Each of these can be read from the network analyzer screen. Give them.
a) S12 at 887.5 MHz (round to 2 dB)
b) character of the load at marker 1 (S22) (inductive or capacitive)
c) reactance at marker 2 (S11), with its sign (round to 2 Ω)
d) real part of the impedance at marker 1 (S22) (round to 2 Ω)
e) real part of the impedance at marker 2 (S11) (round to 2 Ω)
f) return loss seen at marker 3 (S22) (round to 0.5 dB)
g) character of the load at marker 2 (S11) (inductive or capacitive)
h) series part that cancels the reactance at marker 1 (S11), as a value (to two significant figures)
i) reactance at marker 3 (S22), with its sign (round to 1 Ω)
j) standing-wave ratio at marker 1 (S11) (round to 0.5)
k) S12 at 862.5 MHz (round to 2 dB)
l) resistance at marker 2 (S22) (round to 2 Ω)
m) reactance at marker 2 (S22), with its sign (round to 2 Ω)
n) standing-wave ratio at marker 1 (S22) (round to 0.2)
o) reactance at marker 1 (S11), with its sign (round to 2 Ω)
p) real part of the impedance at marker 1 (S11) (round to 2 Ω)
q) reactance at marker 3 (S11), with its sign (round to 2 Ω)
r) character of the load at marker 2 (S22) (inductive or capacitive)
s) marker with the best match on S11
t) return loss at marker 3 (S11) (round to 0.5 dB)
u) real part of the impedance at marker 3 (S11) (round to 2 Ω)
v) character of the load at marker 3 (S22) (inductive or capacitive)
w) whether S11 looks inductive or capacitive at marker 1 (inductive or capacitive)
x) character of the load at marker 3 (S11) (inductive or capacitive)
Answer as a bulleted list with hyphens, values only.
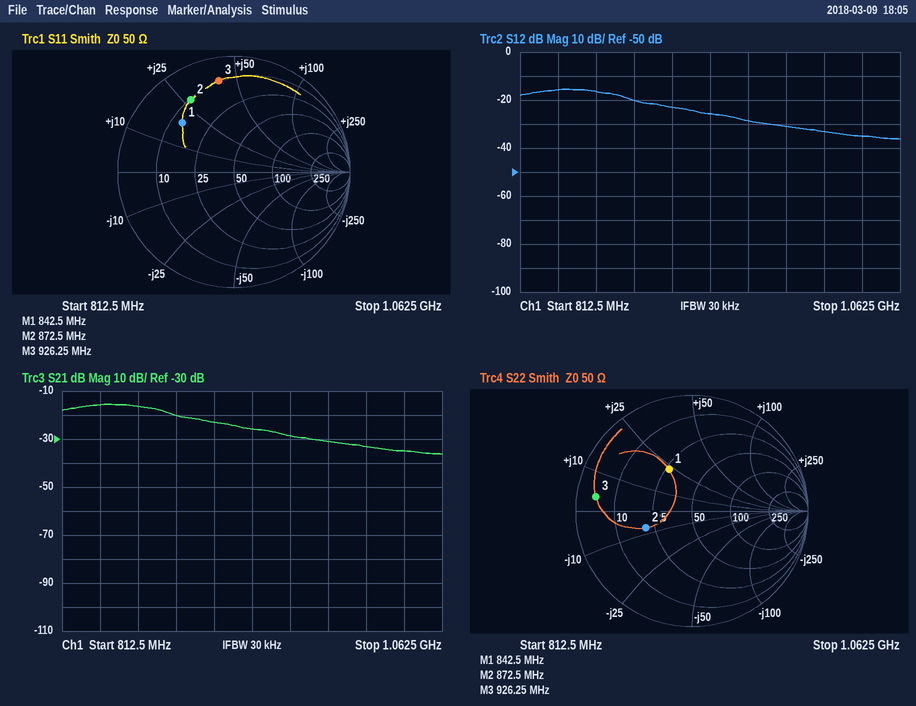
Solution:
- -20 dB
- inductive
- +28 Ω
- 26 Ω
- 10 Ω
- 1.5 dB
- inductive
- 10 pF
- +4 Ω
- 4.0
- -16 dB
- 20 Ω
- -8 Ω
- 2.4
- +18 Ω
- 14 Ω
- +42 Ω
- capacitive
- marker 1
- 2.0 dB
- 10 Ω
- inductive
- inductive
- inductive
